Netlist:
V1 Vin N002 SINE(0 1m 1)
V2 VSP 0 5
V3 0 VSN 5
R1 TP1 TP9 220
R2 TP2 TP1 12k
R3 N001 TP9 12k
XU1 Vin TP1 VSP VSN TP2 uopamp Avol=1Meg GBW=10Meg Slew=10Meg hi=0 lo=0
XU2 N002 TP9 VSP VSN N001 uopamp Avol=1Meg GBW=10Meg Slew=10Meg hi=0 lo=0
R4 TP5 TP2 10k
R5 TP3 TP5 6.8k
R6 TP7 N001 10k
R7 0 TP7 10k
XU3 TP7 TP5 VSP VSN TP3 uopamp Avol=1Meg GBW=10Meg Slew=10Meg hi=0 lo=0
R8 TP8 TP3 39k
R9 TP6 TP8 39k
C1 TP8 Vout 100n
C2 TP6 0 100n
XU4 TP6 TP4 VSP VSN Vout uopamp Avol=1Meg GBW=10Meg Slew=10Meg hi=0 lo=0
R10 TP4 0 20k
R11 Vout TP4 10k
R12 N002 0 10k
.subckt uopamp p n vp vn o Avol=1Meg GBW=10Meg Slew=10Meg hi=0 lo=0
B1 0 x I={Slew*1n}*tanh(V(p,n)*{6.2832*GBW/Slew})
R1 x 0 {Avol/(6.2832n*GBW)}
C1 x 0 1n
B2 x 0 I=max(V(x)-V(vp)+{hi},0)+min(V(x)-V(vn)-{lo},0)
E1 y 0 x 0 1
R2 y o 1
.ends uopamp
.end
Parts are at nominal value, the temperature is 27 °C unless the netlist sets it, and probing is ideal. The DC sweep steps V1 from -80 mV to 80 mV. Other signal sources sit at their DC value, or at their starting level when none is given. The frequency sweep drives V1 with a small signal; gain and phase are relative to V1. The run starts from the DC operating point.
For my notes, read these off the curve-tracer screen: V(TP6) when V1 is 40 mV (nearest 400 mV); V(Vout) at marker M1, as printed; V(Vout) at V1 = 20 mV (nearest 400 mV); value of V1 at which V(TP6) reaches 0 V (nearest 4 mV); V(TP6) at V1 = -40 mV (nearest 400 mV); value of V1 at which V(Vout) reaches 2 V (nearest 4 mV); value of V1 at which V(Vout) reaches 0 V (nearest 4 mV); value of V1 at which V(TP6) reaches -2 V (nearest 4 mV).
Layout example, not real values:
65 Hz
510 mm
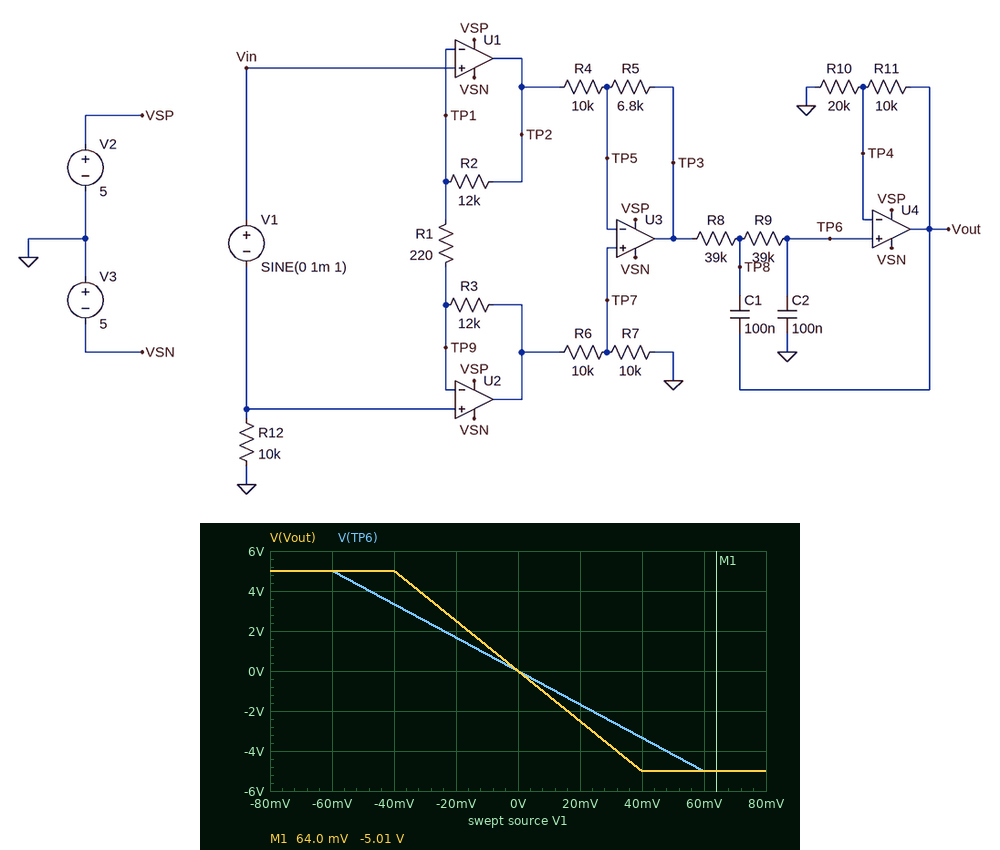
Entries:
-3.2 V
-5.01 V
-2.4 V
0 V
3.2 V
-16 mV
0 V
24 mV
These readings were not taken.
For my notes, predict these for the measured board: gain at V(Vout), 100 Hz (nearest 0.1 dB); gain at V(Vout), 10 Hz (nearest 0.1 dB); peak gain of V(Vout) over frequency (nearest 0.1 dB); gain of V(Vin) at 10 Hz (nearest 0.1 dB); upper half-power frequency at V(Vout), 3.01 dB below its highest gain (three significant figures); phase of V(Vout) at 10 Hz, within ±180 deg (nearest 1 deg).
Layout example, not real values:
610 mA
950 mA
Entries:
26.1 dB
41.9 dB
42.0 dB
0 dB
38.3 Hz
159 deg
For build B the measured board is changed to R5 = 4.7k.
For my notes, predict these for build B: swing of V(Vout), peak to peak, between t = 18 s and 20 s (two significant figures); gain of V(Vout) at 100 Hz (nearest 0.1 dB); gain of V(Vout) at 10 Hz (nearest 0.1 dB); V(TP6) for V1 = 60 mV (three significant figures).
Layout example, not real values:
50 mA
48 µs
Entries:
200 mV
24.1 dB
39.9 dB
-3.97 V
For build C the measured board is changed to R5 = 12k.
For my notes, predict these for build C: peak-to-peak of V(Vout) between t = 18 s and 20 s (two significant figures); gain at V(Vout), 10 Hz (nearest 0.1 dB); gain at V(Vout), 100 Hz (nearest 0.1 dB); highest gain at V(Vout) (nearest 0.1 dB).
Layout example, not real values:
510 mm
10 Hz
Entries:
380 mV
45.5 dB
29.7 dB
45.6 dB
